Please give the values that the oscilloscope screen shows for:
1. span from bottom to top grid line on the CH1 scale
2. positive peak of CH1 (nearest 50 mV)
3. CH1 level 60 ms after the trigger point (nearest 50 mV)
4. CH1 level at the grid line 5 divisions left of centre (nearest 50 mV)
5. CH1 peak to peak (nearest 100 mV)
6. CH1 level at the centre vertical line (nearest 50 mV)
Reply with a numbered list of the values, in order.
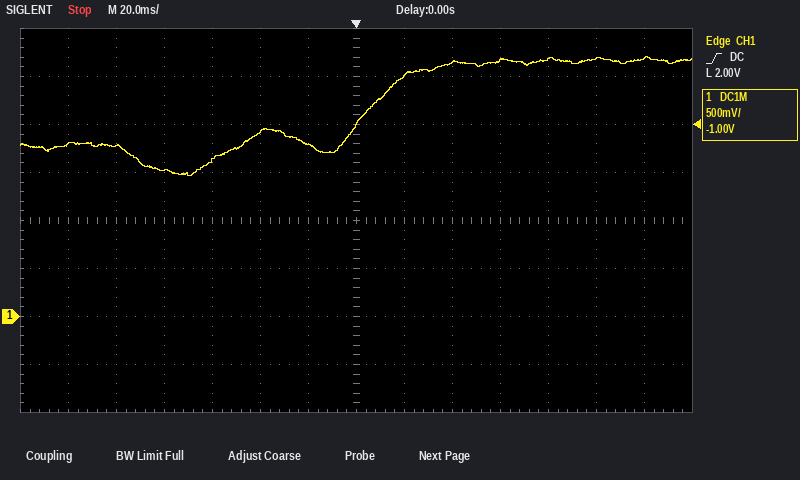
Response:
1. 4 V
2. 2.70 V
3. 2.65 V
4. 1.80 V
5. 1.20 V
6. 2.00 V
